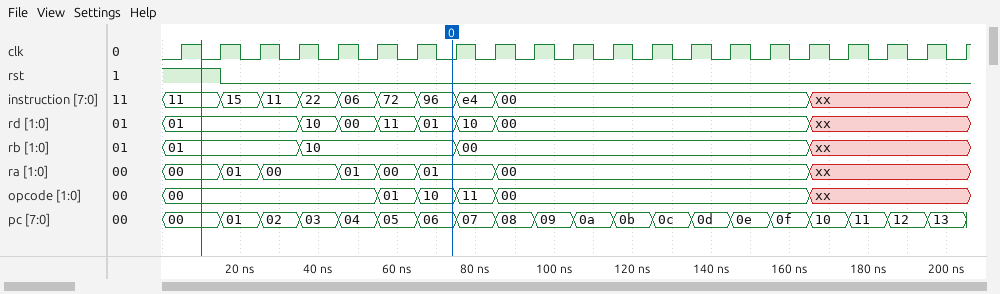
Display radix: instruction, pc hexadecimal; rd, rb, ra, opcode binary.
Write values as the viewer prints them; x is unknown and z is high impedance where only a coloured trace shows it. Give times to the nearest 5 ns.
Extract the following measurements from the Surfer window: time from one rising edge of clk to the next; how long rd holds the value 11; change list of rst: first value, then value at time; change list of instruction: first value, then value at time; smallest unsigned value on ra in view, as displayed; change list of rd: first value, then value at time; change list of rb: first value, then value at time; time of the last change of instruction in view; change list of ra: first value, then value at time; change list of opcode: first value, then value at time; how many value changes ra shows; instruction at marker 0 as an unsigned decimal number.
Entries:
10 ns
10 ns
1, 0 at 15 ns
11, 15 at 15 ns, 11 at 25 ns, 22 at 35 ns, 06 at 45 ns, 72 at 55 ns, 96 at 65 ns, e4 at 75 ns, 00 at 85 ns, xx at 165 ns
00
01, 10 at 35 ns, 00 at 45 ns, 11 at 55 ns, 01 at 65 ns, 10 at 75 ns, 00 at 85 ns, xx at 165 ns
01, 10 at 35 ns, 00 at 75 ns, xx at 165 ns
165 ns
00, 01 at 15 ns, 00 at 25 ns, 01 at 45 ns, 00 at 55 ns, 01 at 65 ns, 00 at 85 ns, xx at 165 ns
00, 01 at 55 ns, 10 at 65 ns, 11 at 75 ns, 00 at 85 ns, xx at 165 ns
7
150
